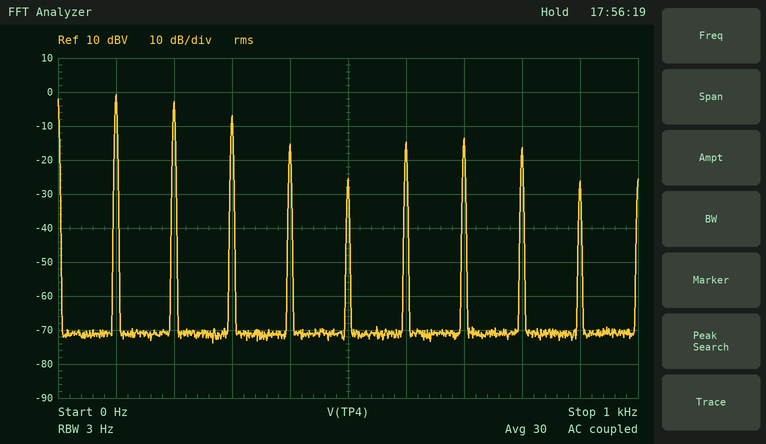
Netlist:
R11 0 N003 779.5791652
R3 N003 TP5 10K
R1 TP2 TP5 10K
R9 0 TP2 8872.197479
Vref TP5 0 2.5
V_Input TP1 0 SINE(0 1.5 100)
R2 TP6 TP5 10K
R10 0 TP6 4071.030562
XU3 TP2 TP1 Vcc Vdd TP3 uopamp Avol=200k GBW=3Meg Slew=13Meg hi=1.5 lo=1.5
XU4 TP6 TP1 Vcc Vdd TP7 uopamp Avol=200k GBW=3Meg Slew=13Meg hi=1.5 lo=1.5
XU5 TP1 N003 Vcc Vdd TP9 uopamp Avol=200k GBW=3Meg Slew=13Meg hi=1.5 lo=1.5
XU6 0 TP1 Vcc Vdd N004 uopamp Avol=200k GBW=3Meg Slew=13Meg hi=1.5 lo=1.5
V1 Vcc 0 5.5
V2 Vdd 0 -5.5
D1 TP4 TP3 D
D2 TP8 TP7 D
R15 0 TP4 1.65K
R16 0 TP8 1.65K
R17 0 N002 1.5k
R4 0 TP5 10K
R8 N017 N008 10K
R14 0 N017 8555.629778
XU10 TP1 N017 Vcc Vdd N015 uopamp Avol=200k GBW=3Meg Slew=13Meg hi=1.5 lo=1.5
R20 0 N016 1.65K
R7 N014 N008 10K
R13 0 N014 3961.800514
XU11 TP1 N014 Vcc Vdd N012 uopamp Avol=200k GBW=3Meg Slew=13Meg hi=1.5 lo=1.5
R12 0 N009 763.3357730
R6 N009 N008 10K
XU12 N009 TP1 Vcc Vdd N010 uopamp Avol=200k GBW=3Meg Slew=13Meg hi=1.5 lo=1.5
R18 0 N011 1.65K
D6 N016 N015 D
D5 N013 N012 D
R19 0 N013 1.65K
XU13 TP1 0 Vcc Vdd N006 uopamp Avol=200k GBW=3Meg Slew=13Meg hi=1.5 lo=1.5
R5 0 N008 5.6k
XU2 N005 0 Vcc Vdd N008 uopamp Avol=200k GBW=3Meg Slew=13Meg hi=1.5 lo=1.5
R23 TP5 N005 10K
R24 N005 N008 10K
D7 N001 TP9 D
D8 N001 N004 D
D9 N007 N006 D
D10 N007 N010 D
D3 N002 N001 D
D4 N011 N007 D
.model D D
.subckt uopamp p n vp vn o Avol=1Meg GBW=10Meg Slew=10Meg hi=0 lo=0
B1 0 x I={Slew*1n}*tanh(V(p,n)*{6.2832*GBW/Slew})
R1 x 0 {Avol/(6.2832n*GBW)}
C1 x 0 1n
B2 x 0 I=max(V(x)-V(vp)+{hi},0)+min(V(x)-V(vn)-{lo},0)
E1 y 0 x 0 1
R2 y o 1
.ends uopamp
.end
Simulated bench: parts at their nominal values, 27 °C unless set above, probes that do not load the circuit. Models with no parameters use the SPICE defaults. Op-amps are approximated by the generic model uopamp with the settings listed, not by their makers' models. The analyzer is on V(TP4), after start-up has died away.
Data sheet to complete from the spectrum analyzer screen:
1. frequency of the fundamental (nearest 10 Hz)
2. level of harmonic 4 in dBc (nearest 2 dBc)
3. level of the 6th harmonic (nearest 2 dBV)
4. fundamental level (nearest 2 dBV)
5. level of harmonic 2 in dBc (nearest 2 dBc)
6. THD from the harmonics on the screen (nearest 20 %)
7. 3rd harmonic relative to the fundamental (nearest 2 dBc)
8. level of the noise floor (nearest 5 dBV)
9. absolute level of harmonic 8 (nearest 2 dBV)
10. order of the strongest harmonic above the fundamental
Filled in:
100 Hz
-14 dBc
-14 dBV
0 dBV
-2 dBc
100 %
-6 dBc
-70 dBV
-16 dBV
2
